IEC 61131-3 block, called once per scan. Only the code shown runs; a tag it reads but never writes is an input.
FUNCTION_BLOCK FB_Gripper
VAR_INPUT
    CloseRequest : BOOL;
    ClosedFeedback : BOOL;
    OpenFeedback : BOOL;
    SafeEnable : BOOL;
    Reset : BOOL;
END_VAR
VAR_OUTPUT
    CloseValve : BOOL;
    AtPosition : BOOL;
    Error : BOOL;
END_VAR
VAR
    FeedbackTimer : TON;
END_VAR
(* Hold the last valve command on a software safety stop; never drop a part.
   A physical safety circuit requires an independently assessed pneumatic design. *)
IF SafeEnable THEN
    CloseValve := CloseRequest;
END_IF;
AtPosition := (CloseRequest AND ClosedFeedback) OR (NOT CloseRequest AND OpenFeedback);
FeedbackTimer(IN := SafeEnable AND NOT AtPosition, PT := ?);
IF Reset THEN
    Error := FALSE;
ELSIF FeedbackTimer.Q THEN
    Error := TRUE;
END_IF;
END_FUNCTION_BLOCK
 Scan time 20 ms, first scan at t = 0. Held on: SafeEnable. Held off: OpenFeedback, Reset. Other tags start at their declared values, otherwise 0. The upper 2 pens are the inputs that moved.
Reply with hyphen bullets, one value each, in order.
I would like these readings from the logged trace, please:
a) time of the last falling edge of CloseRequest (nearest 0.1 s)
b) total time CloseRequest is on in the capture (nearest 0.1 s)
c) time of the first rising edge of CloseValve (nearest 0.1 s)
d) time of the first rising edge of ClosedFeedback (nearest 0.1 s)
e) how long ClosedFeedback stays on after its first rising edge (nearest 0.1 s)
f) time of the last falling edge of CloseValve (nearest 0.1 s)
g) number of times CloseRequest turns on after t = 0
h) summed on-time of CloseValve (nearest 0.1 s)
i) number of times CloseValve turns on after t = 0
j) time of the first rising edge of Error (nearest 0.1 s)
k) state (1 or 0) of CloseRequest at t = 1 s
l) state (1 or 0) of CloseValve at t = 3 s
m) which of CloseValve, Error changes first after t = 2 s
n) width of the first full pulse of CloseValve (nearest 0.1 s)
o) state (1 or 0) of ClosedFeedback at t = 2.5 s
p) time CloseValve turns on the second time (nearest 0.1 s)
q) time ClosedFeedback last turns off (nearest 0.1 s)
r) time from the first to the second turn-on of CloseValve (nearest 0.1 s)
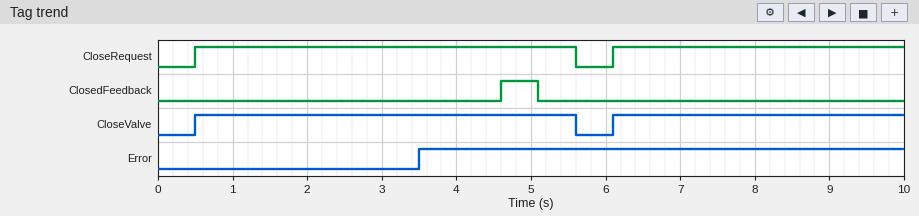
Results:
- 5.6 s
- 9.0 s
- 0.5 s
- 4.6 s
- 0.5 s
- 5.6 s
- 2
- 9.0 s
- 2
- 3.5 s
- 1
- 1
- Error
- 5.1 s
- 0
- 6.1 s
- 5.1 s
- 5.6 s
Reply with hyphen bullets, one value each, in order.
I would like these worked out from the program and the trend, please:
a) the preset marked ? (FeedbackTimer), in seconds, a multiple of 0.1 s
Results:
- 3.5 s
